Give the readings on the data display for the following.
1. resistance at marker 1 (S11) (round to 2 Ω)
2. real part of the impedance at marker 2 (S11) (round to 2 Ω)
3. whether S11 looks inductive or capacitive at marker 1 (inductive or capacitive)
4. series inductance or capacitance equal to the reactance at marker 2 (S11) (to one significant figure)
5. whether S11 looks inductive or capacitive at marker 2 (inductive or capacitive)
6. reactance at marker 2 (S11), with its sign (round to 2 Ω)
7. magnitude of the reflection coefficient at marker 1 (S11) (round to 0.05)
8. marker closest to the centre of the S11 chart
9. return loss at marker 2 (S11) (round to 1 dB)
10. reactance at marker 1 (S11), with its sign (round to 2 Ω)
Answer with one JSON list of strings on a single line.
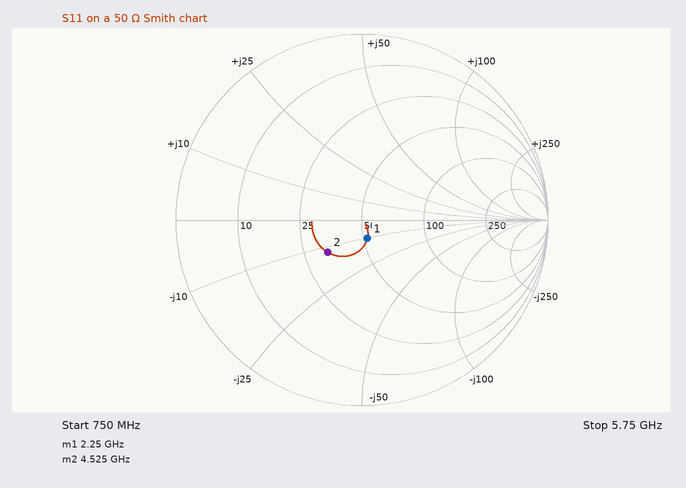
["52 Ω", "32 Ω", "capacitive", "3 pF", "capacitive", "-12 Ω", "0.10", "marker 1", "12 dB", "-10 Ω"]
